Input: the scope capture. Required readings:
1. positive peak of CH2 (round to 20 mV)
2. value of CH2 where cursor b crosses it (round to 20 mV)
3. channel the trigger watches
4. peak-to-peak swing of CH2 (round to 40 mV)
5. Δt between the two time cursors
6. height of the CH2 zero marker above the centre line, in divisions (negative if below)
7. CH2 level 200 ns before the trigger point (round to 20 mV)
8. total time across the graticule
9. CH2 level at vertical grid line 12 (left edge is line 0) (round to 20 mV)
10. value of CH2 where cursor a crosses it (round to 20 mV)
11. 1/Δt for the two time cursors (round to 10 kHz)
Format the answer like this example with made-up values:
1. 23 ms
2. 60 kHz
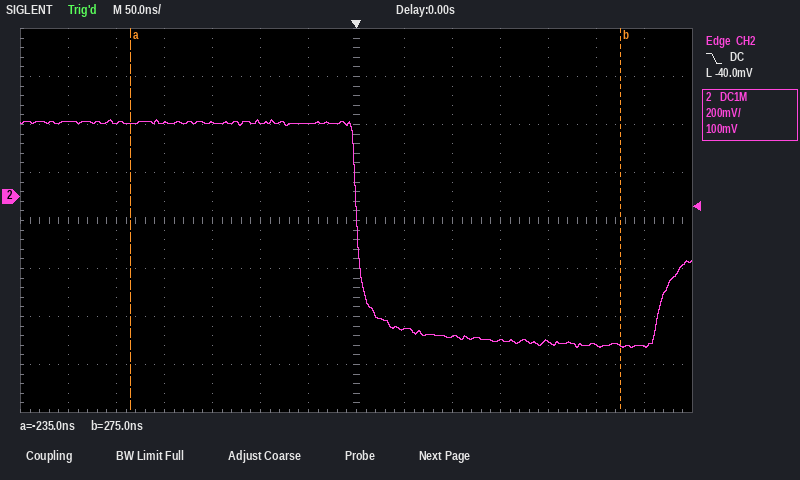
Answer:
1. 320 mV
2. -620 mV
3. CH2
4. 960 mV
5. 510 ns
6. +0.5 div
7. 300 mV
8. 700 ns
9. -620 mV
10. 300 mV
11. 1.96 MHz
